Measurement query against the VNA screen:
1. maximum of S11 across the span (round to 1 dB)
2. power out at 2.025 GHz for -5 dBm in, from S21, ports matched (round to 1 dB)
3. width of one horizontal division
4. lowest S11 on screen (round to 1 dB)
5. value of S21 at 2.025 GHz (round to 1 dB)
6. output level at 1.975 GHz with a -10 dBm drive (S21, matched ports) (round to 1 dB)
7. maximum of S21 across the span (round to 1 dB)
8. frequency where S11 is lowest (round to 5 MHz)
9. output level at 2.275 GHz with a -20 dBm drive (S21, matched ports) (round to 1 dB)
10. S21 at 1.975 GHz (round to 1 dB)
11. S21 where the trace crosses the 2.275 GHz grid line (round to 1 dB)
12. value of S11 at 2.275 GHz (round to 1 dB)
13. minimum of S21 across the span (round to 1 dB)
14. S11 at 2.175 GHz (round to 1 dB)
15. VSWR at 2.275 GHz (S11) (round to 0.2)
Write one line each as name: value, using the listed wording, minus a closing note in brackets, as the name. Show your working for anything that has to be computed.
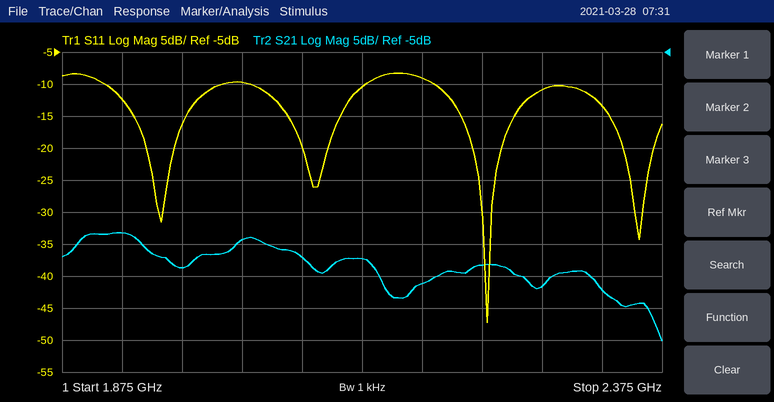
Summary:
maximum of S11 across the span: -8 dB
power out at 2.025 GHz for -5 dBm in, from S21, ports matched: -5 dBm + (-34 dB) = -39 dBm
width of one horizontal division: 50 MHz
lowest S11 on screen: -47 dB
value of S21 at 2.025 GHz: -34 dB
output level at 1.975 GHz with a -10 dBm drive (S21, matched ports): -10 dBm + (-39 dB) = -49 dBm
maximum of S21 across the span: -33 dB
frequency where S11 is lowest: 2.230 GHz
output level at 2.275 GHz with a -20 dBm drive (S21, matched ports): -20 dBm + (-42 dB) = -62 dBm
S21 at 1.975 GHz: -39 dB
S21 where the trace crosses the 2.275 GHz grid line: -42 dB
value of S11 at 2.275 GHz: -11 dB
minimum of S21 across the span: -50 dB
S11 at 2.175 GHz: -9 dB
VSWR at 2.275 GHz (S11): |Γ| = 10^(-11/20) = 0.2818; VSWR = (1 + 0.2818)/(1 − 0.2818) ≈ 1.8
